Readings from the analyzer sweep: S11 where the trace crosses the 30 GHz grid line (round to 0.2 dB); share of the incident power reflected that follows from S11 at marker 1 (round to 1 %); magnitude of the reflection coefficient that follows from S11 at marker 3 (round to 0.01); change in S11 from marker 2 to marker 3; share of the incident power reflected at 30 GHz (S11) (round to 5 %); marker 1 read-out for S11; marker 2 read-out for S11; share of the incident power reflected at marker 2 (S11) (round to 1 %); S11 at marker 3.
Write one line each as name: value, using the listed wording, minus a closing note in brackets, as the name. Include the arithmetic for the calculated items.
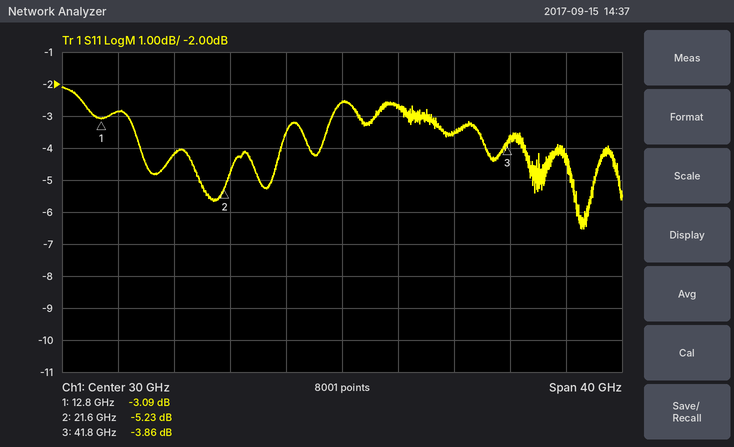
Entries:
S11 where the trace crosses the 30 GHz grid line: -2.6 dB
share of the incident power reflected that follows from S11 at marker 1: 10^(-3.09/10) ≈ 49 %
magnitude of the reflection coefficient that follows from S11 at marker 3: 10^(-3.86/20) ≈ 0.64
change in S11 from marker 2 to marker 3: -3.86 − (-5.23) = 1.37 dB
share of the incident power reflected at 30 GHz (S11): 10^(-2.6/10) ≈ 55 %
marker 1 read-out for S11: -3.09 dB
marker 2 read-out for S11: -5.23 dB
share of the incident power reflected at marker 2 (S11): 10^(-5.23/10) ≈ 30 %
S11 at marker 3: -3.86 dB
